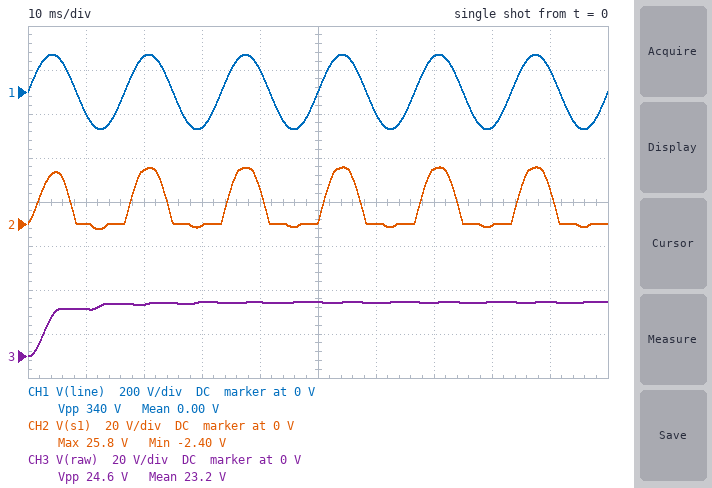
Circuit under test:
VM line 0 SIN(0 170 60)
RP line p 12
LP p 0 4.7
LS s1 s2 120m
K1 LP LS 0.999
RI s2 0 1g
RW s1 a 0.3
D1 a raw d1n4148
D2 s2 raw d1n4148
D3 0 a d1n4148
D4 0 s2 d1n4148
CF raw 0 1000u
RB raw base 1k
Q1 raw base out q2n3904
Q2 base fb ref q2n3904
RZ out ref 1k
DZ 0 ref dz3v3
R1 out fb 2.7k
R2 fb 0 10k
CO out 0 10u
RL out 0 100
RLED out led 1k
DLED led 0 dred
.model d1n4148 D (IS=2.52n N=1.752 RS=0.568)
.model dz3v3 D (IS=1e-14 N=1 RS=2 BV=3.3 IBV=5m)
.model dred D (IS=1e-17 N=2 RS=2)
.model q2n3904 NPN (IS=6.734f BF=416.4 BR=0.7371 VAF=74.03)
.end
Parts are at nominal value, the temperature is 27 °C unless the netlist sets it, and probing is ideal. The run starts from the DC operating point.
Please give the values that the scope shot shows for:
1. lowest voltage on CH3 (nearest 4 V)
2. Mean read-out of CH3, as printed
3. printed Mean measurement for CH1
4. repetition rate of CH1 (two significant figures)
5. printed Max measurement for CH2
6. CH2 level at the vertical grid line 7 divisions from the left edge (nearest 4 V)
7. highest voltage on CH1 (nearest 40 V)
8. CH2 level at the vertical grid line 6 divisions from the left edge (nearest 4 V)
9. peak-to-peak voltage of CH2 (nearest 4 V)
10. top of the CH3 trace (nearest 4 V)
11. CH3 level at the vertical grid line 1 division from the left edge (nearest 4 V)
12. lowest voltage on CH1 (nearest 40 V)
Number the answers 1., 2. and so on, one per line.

1. 0 V
2. 23.2 V
3. 0.00 V
4. 60 Hz
5. 25.8 V
6. 24 V
7. 160 V
8. 0 V
9. 28 V
10. 24 V
11. 20 V
12. -160 V
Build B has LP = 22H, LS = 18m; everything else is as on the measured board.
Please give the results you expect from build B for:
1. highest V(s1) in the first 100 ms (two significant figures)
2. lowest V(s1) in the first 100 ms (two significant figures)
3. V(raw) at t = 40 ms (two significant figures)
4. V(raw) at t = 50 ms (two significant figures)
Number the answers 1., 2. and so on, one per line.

1. 4.0 V
2. -1.1 V
3. 3.1 V
4. 3.0 V
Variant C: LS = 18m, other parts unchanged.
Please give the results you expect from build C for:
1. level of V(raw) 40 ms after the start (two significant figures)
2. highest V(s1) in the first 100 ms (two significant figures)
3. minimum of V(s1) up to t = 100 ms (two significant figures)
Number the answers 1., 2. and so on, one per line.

1. 8.3 V
2. 9.4 V
3. -1.5 V
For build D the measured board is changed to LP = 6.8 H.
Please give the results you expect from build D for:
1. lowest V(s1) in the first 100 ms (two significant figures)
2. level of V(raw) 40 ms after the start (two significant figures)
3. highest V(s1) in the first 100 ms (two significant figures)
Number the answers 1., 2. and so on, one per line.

1. -2.1 V
2. 20 V
3. 21 V
